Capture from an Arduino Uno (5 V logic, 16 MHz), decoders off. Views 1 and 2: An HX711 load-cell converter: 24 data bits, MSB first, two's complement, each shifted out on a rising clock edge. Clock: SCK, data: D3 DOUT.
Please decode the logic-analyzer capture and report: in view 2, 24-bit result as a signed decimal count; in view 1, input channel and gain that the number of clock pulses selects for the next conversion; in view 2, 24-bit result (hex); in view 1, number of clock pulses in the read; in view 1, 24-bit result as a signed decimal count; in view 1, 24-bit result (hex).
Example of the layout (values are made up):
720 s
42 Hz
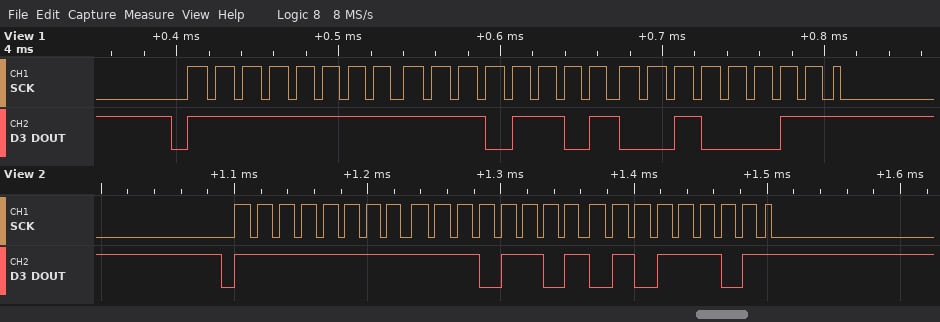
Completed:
-4771
channel A, gain 128
0xFFED5D
25
-4829
0xFFED23
